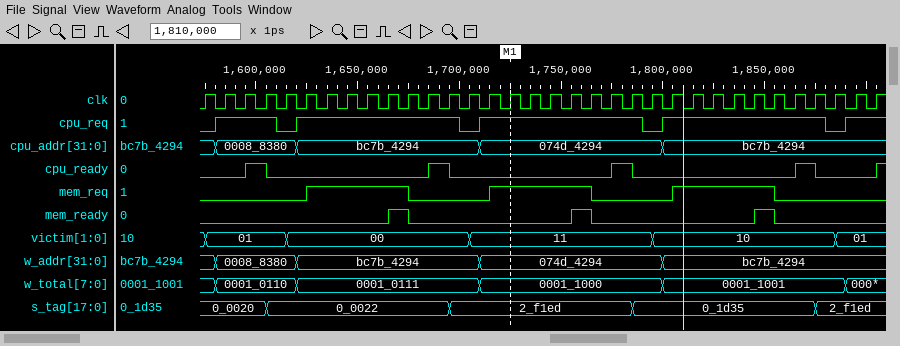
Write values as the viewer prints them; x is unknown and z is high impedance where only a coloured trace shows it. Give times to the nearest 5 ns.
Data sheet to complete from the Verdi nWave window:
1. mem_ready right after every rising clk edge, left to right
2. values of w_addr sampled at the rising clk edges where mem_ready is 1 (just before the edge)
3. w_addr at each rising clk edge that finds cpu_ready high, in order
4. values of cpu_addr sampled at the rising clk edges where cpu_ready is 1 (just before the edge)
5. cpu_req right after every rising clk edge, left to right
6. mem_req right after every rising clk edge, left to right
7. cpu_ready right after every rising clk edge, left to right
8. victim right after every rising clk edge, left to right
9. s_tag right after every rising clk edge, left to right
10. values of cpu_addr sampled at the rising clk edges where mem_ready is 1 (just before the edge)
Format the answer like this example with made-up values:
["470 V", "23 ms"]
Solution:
["0 0 0 0 0 0 0 0 0 1 0 0 0 0 0 0 0 0 1 0 0 0 0 0 0 0 0 1 0 0 0 0 0 0", "bc7b_4294, 074d_4294, bc7b_4294", "0008_8380, bc7b_4294, 074d_4294, bc7b_4294", "0008_8380, bc7b_4294, 074d_4294, bc7b_4294", "0 1 1 1 0 1 1 1 1 1 1 1 1 0 1 1 1 1 1 1 1 1 0 1 1 1 1 1 1 1 1 0 1 1", "0 0 0 0 0 1 1 1 1 1 0 0 0 0 1 1 1 1 1 0 0 0 0 1 1 1 1 1 0 0 0 0 0 0", "0 0 1 0 0 0 0 0 0 0 0 1 0 0 0 0 0 0 0 0 1 0 0 0 0 0 0 0 0 1 0 0 0 1", "01, 01, 01, 01, 00, 00, 00, 00, 00, 00, 00, 00, 00, 11, 11, 11, 11, 11, 11, 11, 11, 11, 10, 10, 10, 10, 10, 10, 10, 10, 10, 01, 01, 01", "0_0020, 0_0020, 0_0020, 0_0022, 0_0022, 0_0022, 0_0022, 0_0022, 0_0022, 0_0022, 0_0022, 0_0022, 2_f1ed, 2_f1ed, 2_f1ed, 2_f1ed, 2_f1ed, 2_f1ed, 2_f1ed, 2_f1ed, 2_f1ed, 0_1d35, 0_1d35, 0_1d35, 0_1d35, 0_1d35, 0_1d35, 0_1d35, 0_1d35, 0_1d35, 2_f1ed, 2_f1ed, 2_f1ed, 2_f1ed", "bc7b_4294, 074d_4294, bc7b_4294"]
